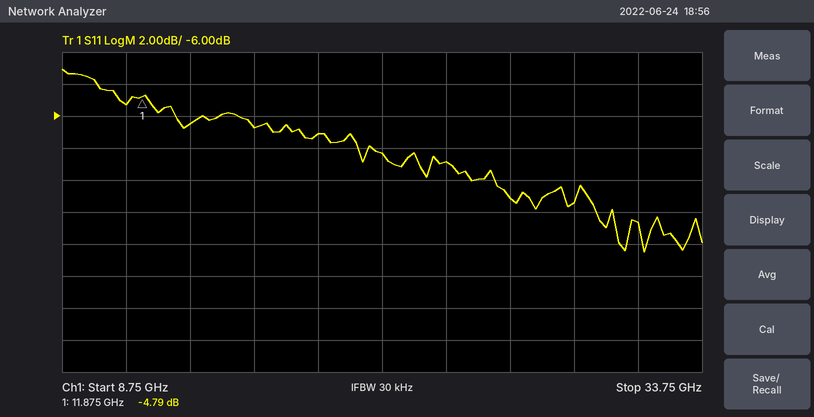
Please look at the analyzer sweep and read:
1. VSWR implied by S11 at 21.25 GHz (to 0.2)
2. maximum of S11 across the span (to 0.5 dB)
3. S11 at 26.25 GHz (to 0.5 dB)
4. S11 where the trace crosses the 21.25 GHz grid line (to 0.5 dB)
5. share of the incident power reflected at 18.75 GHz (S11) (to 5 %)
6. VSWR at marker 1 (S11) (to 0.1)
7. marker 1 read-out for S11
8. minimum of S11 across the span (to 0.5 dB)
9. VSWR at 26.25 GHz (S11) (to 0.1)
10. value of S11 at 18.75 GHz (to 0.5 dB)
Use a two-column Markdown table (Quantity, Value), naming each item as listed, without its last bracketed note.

| Quantity | Value |
|---|---|
| VSWR implied by S11 at 21.25 GHz | 2.2 |
| maximum of S11 across the span | -3.0 dB |
| S11 at 26.25 GHz | -11.0 dB |
| S11 where the trace crosses the 21.25 GHz grid line | -8.5 dB |
| share of the incident power reflected at 18.75 GHz (S11) | 20 % |
| VSWR at marker 1 (S11) | 3.7 |
| marker 1 read-out for S11 | -4.79 dB |
| minimum of S11 across the span | -14.5 dB |
| VSWR at 26.25 GHz (S11) | 1.8 |
| value of S11 at 18.75 GHz | -7.0 dB |
